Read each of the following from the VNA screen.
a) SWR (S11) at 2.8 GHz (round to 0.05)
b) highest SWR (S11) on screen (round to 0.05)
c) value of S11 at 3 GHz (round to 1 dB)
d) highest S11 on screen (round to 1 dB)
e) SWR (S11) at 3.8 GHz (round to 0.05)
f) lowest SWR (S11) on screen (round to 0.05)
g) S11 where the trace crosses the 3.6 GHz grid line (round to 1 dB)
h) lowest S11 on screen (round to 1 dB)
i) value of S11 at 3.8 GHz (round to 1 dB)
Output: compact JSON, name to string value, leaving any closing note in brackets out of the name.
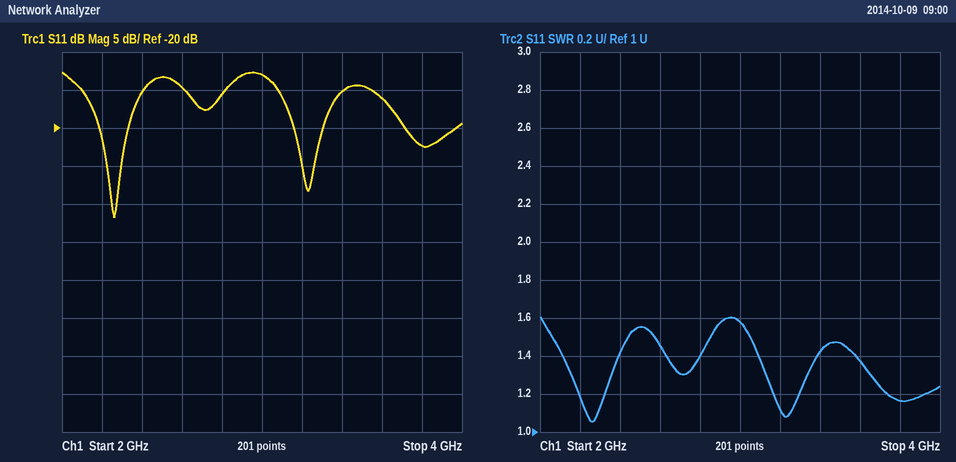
{"SWR (S11) at 2.8 GHz": "1.40", "highest SWR (S11) on screen": "1.60", "value of S11 at 3 GHz": "-13 dB", "highest S11 on screen": "-13 dB", "SWR (S11) at 3.8 GHz": "1.15", "lowest SWR (S11) on screen": "1.05", "S11 where the trace crosses the 3.6 GHz grid line": "-16 dB", "lowest S11 on screen": "-32 dB", "value of S11 at 3.8 GHz": "-22 dB"}
